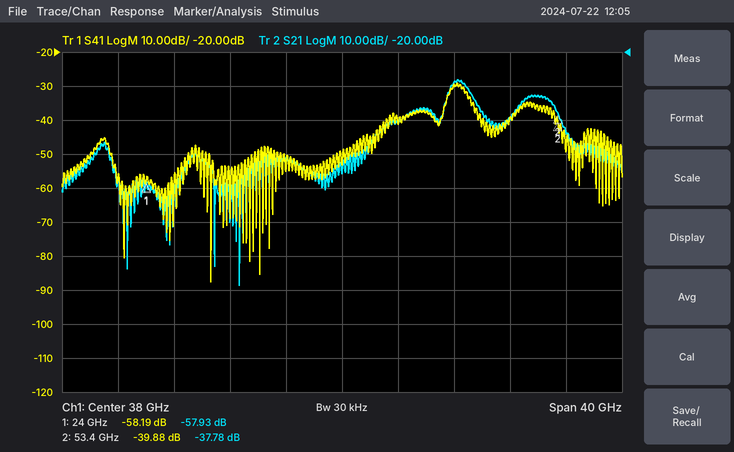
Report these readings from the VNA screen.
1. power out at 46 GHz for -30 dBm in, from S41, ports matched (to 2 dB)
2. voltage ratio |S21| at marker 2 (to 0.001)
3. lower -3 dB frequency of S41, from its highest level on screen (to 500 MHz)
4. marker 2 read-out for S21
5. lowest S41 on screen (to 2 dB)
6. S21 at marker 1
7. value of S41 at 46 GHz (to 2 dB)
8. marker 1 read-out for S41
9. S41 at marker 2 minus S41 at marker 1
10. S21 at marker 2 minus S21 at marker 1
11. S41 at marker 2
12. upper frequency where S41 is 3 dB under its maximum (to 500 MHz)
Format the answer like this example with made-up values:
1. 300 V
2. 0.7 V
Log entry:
1. -60 dBm
2. 0.013
3. 45.5 GHz
4. -37.78 dB
5. -88 dB
6. -57.93 dB
7. -30 dB
8. -58.19 dB
9. 18.31 dB
10. 20.15 dB
11. -39.88 dB
12. 47.0 GHz
